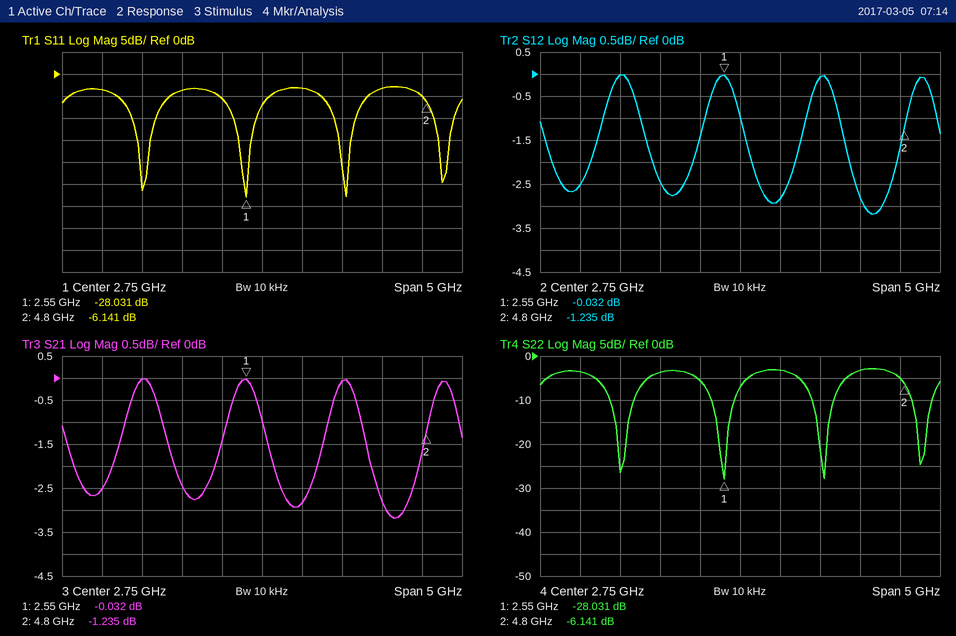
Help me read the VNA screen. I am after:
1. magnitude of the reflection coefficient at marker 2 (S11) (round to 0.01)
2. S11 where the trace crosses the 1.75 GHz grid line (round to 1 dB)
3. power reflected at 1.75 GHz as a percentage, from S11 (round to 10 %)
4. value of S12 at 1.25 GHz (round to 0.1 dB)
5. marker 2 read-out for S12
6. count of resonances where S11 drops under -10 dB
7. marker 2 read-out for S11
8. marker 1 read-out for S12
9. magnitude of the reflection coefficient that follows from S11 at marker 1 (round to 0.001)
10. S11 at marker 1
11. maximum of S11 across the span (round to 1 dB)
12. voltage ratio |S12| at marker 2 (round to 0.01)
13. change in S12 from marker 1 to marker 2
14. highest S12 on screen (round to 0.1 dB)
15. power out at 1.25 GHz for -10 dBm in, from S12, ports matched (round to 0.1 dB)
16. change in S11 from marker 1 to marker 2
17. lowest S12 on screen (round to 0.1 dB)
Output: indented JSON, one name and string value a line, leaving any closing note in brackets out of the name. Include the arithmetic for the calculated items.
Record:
{
  "magnitude of the reflection coefficient at marker 2 (S11)": "10^(-6.141/20) ≈ 0.49",
  "S11 where the trace crosses the 1.75 GHz grid line": "-4 dB",
  "power reflected at 1.75 GHz as a percentage, from S11": "10^(-4/10) ≈ 40 %",
  "value of S12 at 1.25 GHz": "0.0 dB",
  "marker 2 read-out for S12": "-1.235 dB",
  "count of resonances where S11 drops under -10 dB": "4",
  "marker 2 read-out for S11": "-6.141 dB",
  "marker 1 read-out for S12": "-0.032 dB",
  "magnitude of the reflection coefficient that follows from S11 at marker 1": "10^(-28.031/20) ≈ 0.040",
  "S11 at marker 1": "-28.031 dB",
  "maximum of S11 across the span": "-3 dB",
  "voltage ratio |S12| at marker 2": "10^(-1.235/20) ≈ 0.87",
  "change in S12 from marker 1 to marker 2": "-1.235 − (-0.032) = -1.203 dB",
  "highest S12 on screen": "0.0 dB",
  "power out at 1.25 GHz for -10 dBm in, from S12, ports matched": "-10 dBm + (0.0 dB) = -10.0 dBm",
  "change in S11 from marker 1 to marker 2": "-6.141 − (-28.031) = 21.890 dB",
  "lowest S12 on screen": "-3.2 dB"
}
